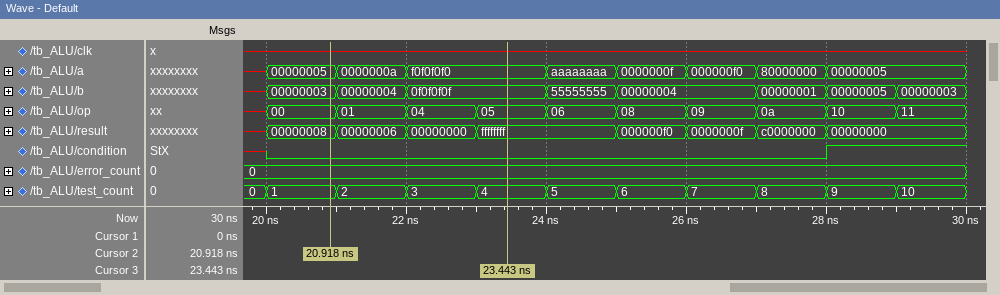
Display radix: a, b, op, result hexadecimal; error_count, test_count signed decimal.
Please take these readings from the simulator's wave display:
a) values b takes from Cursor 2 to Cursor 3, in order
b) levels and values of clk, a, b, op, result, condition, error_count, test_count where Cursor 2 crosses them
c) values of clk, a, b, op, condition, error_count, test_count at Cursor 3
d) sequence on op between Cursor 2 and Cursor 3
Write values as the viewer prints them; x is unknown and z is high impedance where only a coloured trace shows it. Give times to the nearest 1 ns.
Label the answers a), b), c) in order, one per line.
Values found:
a) 00000003, 00000004, 0f0f0f0f
b) clk=x, a=00000005, b=00000003, op=00, result=00000008, condition=0, error_count=0, test_count=1
c) clk=x, a=f0f0f0f0, b=0f0f0f0f, op=05, condition=0, error_count=0, test_count=4
d) 00, 01, 04, 05
